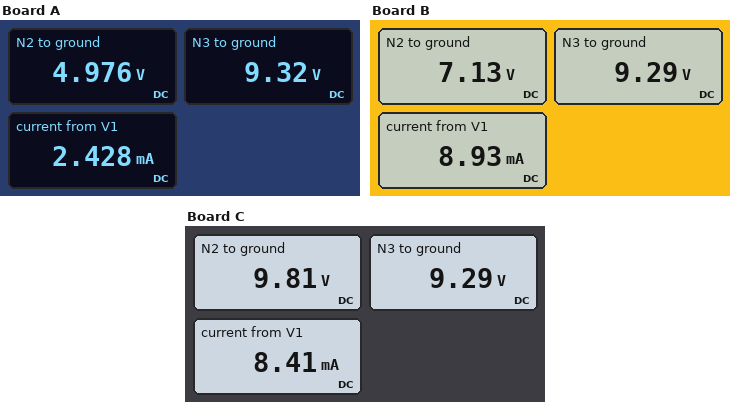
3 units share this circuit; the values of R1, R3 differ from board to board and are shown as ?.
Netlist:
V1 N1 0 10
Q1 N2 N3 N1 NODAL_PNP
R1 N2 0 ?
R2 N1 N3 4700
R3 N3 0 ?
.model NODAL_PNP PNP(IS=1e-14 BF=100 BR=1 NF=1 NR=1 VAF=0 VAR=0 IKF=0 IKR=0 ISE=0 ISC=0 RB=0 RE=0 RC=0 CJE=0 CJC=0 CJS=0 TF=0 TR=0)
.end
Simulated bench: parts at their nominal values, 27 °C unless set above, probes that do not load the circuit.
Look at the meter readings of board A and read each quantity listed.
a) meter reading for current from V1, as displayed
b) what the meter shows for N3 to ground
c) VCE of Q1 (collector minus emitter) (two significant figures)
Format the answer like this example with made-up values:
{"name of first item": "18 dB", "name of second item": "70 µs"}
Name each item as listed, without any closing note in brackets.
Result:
{"meter reading for current from V1, as displayed": "2.428 mA", "what the meter shows for N3 to ground": "9.32 V", "VCE of Q1 (collector minus emitter)": "-5.0 V"}
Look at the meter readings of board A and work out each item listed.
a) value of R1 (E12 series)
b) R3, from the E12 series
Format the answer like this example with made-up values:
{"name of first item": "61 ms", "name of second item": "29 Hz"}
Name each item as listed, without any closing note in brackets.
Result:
{"value of R1": "2.2 kΩ", "R3, from the E12 series": "56 kΩ"}
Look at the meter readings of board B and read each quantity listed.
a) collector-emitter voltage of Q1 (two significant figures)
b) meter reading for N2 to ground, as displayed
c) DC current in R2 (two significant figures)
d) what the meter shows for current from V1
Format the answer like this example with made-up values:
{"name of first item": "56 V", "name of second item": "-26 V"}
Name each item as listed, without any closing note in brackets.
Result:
{"collector-emitter voltage of Q1": "-2.9 V", "meter reading for N2 to ground, as displayed": "7.13 V", "DC current in R2": "150 µA", "what the meter shows for current from V1": "8.93 mA"}
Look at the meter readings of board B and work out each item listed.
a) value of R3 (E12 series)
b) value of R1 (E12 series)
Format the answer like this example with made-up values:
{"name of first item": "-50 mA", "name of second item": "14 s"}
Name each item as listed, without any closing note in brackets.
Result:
{"value of R3": "39 kΩ", "value of R1": "820 Ω"}
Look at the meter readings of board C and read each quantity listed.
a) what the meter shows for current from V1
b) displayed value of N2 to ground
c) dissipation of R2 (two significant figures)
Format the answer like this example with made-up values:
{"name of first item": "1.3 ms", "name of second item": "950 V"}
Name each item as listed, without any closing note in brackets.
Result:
{"what the meter shows for current from V1": "8.41 mA", "displayed value of N2 to ground": "9.81 V", "dissipation of R2": "110 µW"}
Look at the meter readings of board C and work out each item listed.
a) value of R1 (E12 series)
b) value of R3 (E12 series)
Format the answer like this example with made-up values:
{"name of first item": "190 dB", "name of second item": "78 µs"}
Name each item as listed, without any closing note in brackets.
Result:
{"value of R1": "1.2 kΩ", "value of R3": "39 kΩ"}
